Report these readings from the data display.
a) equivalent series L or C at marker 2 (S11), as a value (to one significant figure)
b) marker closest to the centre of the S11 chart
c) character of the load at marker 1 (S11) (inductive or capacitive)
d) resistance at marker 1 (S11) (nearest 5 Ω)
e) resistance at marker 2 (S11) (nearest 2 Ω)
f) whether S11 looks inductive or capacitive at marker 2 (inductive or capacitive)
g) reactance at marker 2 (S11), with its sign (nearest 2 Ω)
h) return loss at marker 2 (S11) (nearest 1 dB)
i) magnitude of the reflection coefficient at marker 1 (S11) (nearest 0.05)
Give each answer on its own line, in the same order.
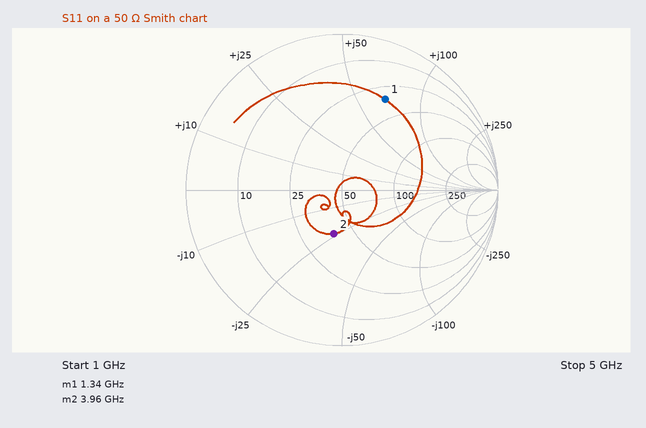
2 pF
marker 2
inductive
35 Ω
38 Ω
capacitive
-24 Ω
11 dB
0.65
